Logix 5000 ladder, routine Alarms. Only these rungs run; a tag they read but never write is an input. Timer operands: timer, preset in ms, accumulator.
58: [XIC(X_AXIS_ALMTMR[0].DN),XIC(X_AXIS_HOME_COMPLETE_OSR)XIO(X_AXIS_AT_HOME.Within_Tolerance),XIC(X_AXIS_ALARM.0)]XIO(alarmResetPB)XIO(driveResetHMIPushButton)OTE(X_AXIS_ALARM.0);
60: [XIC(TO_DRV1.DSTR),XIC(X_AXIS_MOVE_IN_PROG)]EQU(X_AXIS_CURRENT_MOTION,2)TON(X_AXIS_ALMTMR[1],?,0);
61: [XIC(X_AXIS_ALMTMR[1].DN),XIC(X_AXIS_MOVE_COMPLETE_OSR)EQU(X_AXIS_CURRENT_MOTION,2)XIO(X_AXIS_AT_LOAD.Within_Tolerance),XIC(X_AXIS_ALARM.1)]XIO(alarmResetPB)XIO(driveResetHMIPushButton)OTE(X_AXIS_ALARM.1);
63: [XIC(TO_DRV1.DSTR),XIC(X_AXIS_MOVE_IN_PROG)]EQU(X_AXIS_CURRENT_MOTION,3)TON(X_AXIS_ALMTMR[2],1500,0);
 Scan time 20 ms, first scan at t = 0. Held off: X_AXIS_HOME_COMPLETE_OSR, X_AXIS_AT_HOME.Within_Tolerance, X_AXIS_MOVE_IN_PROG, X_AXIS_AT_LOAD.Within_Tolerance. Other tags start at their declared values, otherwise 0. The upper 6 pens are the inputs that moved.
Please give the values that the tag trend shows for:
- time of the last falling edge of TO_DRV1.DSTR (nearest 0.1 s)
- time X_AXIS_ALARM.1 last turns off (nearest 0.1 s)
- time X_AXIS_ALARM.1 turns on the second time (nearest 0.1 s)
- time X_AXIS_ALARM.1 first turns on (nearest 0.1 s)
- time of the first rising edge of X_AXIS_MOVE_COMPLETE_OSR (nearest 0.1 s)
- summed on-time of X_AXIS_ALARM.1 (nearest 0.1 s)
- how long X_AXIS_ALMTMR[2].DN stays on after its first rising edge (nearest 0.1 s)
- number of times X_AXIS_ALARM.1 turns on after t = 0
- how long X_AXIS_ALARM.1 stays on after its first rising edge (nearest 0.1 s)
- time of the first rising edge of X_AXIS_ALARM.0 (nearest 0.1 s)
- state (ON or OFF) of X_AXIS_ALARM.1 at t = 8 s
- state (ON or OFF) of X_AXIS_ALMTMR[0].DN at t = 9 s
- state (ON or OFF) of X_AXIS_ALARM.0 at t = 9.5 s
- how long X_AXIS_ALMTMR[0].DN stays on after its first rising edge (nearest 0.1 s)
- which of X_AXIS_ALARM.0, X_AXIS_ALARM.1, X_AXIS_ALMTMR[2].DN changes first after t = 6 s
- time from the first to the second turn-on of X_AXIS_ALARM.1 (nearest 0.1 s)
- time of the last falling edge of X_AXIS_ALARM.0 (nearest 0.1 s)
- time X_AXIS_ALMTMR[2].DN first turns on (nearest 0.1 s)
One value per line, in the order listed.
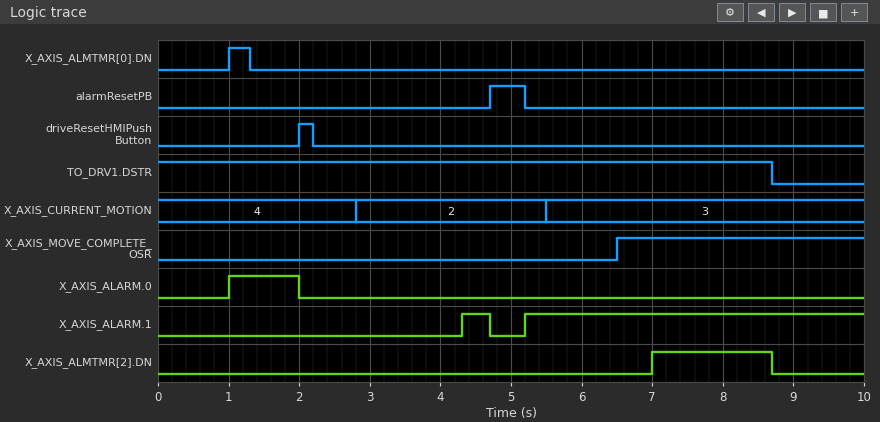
8.7 s
4.7 s
5.2 s
4.3 s
6.5 s
5.2 s
1.7 s
2
0.4 s
1.0 s
ON
OFF
OFF
0.3 s
X_AXIS_ALMTMR[2].DN
0.9 s
2.0 s
7.0 s
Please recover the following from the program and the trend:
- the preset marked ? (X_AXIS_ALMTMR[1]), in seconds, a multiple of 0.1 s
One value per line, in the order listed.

1.5 s
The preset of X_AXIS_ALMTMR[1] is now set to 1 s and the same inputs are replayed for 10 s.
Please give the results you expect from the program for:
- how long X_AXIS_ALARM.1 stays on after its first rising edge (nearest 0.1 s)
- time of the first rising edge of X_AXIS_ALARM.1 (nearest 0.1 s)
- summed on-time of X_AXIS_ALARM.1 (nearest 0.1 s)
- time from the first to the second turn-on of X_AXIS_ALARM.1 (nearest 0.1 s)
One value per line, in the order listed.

0.9 s
3.8 s
5.7 s
1.4 s
